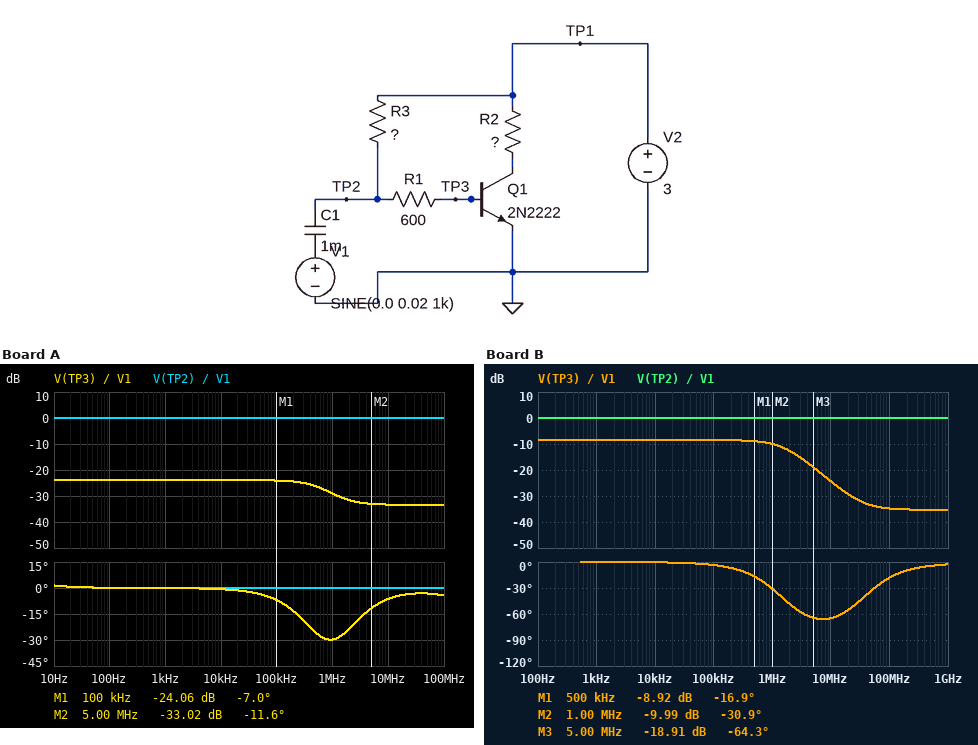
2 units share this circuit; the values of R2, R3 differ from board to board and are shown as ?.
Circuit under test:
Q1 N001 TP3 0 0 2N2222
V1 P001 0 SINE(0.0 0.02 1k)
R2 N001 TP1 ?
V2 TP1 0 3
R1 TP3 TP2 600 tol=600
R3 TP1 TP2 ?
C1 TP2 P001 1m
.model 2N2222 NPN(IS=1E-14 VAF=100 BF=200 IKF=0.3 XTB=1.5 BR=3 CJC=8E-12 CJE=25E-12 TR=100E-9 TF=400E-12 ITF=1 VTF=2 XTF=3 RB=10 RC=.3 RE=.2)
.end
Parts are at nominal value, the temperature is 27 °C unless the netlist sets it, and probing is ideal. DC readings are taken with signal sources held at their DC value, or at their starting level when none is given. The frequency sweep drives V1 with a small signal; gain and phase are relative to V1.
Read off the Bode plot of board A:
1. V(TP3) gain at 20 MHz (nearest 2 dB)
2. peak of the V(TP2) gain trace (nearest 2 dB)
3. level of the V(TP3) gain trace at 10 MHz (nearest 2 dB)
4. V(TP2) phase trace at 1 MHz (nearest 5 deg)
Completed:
-34 dB
0 dB
-34 dB
0 deg
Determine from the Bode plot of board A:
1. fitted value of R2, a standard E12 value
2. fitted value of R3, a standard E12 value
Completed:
330 Ω
39 kΩ
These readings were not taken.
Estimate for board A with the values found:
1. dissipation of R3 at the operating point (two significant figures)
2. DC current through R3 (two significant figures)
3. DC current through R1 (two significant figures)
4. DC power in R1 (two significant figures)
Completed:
130 µW
58 µA
58 µA
2.0 µW
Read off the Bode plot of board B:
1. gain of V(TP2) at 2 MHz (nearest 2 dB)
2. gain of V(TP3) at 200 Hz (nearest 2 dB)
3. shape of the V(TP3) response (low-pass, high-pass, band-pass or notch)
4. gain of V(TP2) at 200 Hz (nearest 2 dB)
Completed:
0 dB
-8 dB
low-pass
0 dB
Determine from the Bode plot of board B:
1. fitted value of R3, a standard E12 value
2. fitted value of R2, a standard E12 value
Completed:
27 kΩ
68 Ω
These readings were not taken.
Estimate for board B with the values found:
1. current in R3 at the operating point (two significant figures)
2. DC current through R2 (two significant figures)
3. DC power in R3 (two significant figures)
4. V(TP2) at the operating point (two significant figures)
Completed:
82 µA
16 mA
180 µW
780 mV
